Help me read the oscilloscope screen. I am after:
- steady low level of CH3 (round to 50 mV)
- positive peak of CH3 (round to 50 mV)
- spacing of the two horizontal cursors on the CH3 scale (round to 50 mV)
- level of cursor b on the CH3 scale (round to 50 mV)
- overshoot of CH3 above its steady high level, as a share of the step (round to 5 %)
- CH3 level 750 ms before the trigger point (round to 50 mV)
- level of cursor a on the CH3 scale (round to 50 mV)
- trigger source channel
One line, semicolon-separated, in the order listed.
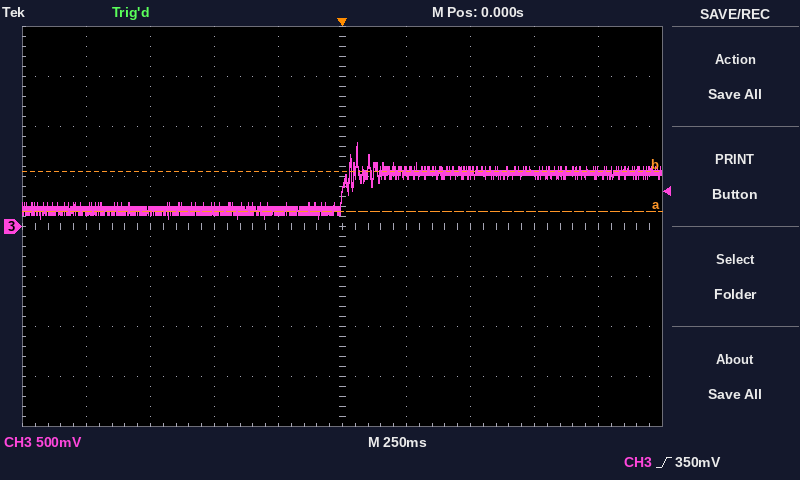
150 mV; 850 mV; 400 mV; 550 mV; 80 %; 150 mV; 150 mV; CH3
